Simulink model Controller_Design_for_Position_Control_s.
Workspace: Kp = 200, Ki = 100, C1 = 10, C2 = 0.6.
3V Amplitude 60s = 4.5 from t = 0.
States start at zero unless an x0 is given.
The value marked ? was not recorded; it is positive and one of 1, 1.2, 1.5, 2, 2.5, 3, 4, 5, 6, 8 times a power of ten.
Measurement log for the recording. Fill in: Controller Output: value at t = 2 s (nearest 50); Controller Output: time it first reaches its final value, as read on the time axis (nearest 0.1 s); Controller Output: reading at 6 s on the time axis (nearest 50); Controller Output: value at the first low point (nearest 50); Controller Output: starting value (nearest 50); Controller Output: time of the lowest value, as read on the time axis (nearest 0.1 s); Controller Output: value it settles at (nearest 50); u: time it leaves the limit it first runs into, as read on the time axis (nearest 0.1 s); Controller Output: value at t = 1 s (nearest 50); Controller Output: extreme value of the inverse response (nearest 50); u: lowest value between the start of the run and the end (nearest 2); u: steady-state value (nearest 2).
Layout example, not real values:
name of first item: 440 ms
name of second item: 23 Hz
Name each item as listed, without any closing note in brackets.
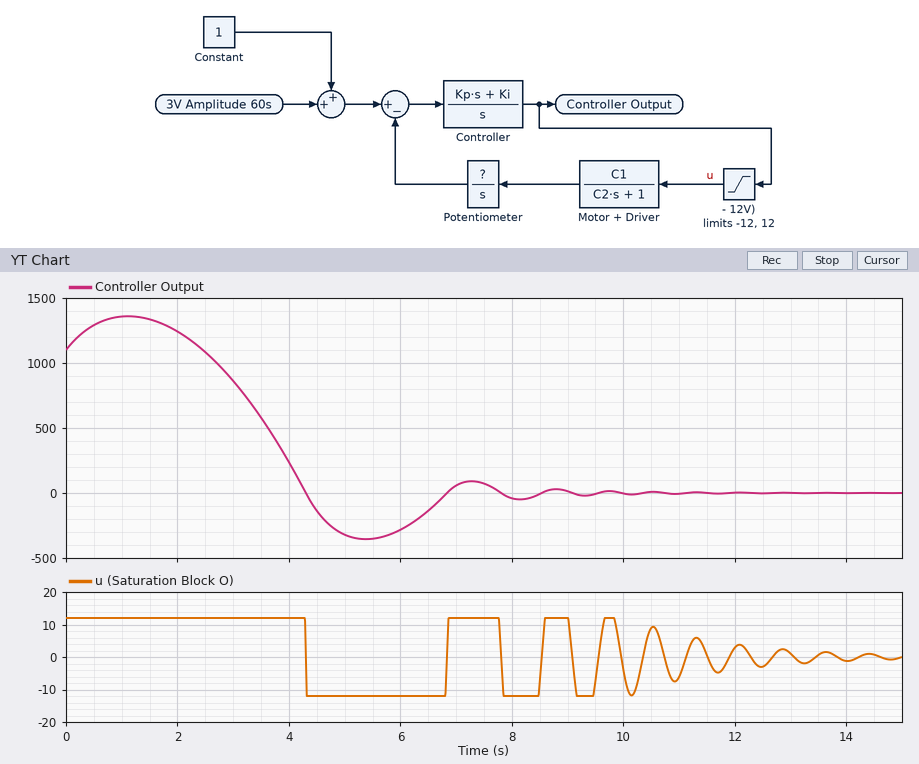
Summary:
Controller Output: value at t = 2 s: 1250
Controller Output: time it first reaches its final value, as read on the time axis: 4.3 s
Controller Output: reading at 6 s on the time axis: -300
Controller Output: value at the first low point: -350
Controller Output: starting value: 1100
Controller Output: time of the lowest value, as read on the time axis: 5.4 s
Controller Output: value it settles at: 0
u: time it leaves the limit it first runs into, as read on the time axis: 4.3 s
Controller Output: value at t = 1 s: 1350
Controller Output: extreme value of the inverse response: 1350
u: lowest value between the start of the run and the end: -12
u: steady-state value: 0
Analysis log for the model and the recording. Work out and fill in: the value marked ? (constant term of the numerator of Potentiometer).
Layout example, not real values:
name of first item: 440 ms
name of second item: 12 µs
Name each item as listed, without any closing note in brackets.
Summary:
the value marked ?: 0.02
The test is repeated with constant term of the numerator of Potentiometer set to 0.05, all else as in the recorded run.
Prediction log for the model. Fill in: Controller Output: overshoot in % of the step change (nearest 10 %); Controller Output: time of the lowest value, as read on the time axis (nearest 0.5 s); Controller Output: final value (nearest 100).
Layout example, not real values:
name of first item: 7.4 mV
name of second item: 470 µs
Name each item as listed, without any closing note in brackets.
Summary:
Controller Output: overshoot in % of the step change: 30 %
Controller Output: time of the lowest value, as read on the time axis: 2.5 s
Controller Output: final value: 0
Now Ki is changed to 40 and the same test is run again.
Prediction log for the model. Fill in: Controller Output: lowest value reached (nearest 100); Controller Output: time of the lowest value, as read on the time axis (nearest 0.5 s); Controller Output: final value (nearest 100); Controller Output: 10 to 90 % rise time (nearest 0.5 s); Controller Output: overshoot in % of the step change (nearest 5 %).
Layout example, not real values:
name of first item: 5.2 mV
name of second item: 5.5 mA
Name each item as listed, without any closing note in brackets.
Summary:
Controller Output: lowest value reached: -100
Controller Output: time of the lowest value, as read on the time axis: 4.0 s
Controller Output: final value: 0
Controller Output: 10 to 90 % rise time: 2.0 s
Controller Output: overshoot in % of the step change: 10 %
